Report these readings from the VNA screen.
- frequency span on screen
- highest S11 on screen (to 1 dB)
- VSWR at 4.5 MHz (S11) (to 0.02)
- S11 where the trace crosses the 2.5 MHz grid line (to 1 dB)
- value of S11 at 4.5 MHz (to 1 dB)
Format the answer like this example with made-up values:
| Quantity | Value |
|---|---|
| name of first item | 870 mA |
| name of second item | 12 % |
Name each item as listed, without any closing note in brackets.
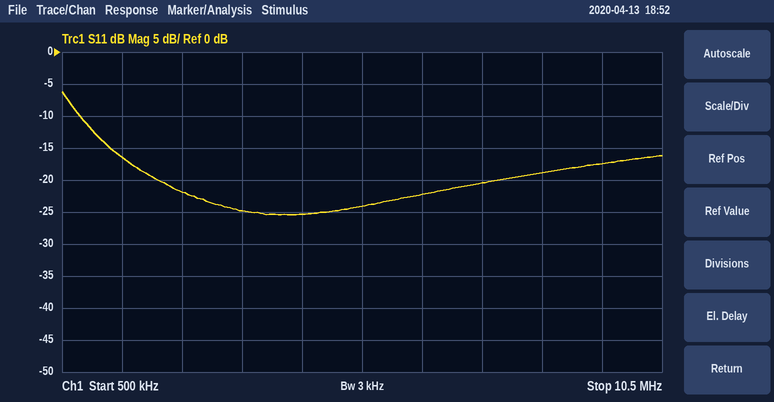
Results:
| Quantity | Value |
|---|---|
| frequency span on screen | 10 MHz |
| highest S11 on screen | -6 dB |
| VSWR at 4.5 MHz (S11) | 1.12 |
| S11 where the trace crosses the 2.5 MHz grid line | -22 dB |
| value of S11 at 4.5 MHz | -25 dB |
